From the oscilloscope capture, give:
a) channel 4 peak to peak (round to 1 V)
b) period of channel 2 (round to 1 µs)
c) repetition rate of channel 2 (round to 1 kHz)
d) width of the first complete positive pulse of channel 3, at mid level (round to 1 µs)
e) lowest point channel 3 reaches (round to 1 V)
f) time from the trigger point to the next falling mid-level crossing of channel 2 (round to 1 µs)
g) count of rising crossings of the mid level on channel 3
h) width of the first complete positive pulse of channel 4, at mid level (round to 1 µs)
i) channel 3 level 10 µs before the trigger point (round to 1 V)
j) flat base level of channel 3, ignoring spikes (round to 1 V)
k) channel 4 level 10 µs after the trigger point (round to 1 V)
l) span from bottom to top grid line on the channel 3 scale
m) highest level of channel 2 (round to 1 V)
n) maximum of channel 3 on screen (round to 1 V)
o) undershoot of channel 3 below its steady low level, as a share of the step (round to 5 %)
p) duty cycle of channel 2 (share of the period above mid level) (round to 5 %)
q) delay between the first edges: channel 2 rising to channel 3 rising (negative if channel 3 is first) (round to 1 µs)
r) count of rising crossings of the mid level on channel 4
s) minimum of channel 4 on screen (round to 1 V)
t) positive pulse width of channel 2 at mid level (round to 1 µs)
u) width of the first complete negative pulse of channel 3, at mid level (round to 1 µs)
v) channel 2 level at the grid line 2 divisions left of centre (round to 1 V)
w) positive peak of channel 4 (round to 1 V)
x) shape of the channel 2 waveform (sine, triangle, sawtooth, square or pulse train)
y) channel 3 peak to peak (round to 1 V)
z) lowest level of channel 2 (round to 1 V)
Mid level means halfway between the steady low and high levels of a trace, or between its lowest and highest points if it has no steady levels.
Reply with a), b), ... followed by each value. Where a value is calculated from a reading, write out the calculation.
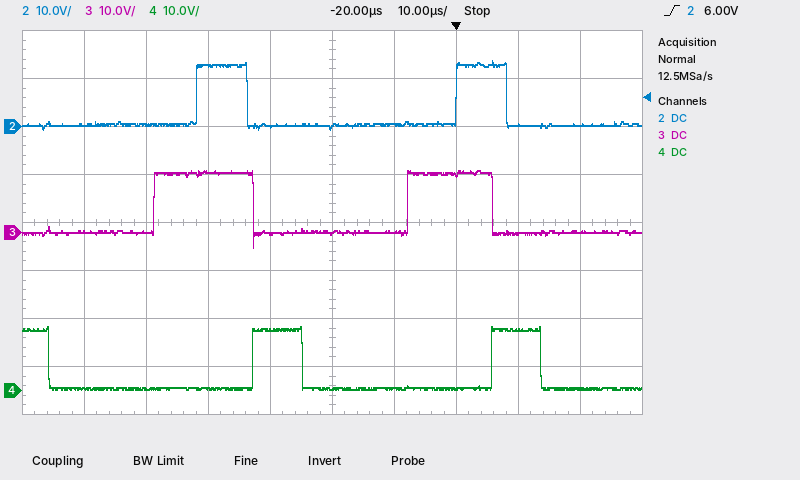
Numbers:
a) 13 V − (0 V) = 13 V
b) 42 µs
c) 1 / 42 µs ≈ 24 kHz
d) 16 µs
e) -3 V
f) 8 µs
g) 2
h) 8 µs
i) 0 V
j) 0 V
k) 13 V
l) 80 V
m) 14 V
n) 13 V
o) 25 %
p) 8 µs / 42 µs ≈ 19.0 %, so 20 % to the nearest 5 %
q) -7 µs
r) 2
s) 0 V
t) 8 µs
u) 25 µs
v) 13 V
w) 13 V
x) pulse train
y) 13 V − (-3 V) = 16 V
z) -1 V
